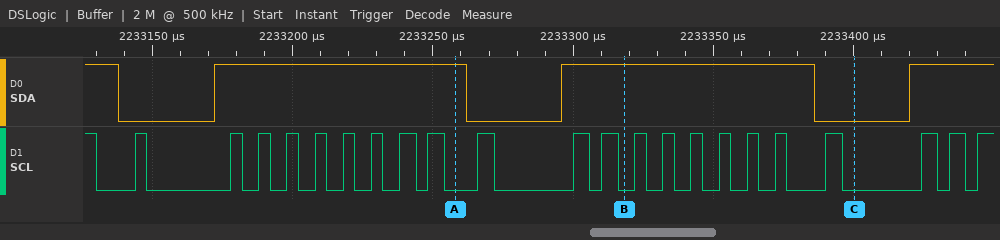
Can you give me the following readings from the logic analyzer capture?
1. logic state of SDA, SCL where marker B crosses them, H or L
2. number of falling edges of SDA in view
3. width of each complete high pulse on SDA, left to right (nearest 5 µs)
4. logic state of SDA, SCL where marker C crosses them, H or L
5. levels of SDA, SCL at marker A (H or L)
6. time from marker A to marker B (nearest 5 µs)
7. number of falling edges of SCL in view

SDA=H, SCL=L
3
90 µs, 90 µs
SDA=L, SCL=L
SDA=H, SCL=L
60 µs
22
